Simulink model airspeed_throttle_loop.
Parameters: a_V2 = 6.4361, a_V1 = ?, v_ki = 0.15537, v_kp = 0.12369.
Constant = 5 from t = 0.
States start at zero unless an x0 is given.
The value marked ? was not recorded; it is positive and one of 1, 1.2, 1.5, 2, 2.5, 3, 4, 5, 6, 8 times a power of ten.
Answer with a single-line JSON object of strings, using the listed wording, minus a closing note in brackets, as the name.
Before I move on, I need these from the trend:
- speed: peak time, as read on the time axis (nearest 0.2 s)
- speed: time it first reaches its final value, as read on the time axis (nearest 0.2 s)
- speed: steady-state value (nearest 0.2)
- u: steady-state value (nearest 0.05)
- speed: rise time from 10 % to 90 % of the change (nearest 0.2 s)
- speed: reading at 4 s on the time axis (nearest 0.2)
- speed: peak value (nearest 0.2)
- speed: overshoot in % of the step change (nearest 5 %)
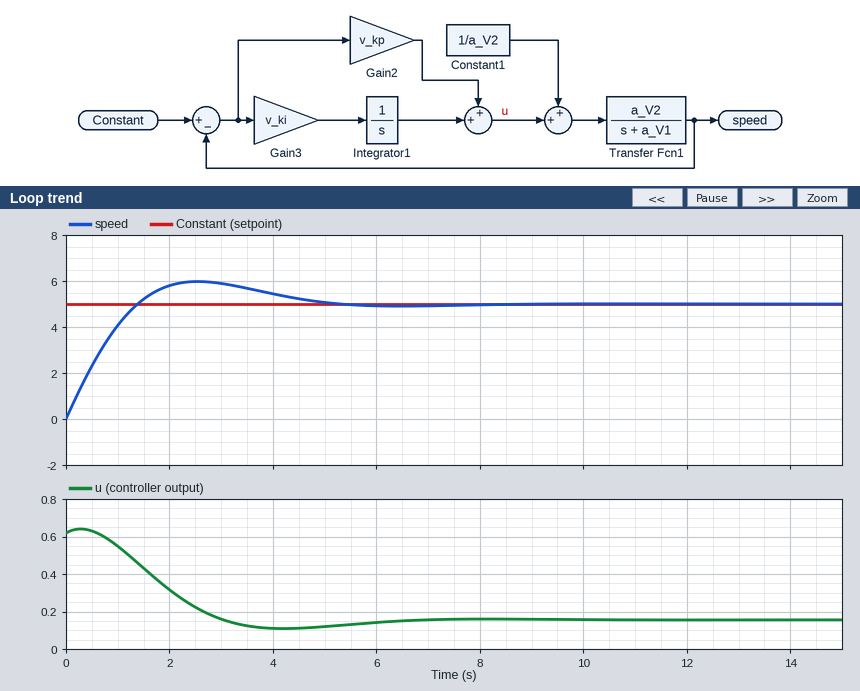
{"speed: peak time, as read on the time axis": "2.6 s", "speed: time it first reaches its final value, as read on the time axis": "1.4 s", "speed: steady-state value": "5.0", "u: steady-state value": "0.15", "speed: rise time from 10 % to 90 % of the change": "1.0 s", "speed: reading at 4 s on the time axis": "5.4", "speed: peak value": "6.0", "speed: overshoot in % of the step change": "20 %"}
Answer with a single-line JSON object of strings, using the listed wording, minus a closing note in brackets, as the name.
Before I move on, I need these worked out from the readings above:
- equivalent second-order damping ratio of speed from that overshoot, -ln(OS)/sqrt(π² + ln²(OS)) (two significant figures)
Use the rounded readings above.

{"equivalent second-order damping ratio of speed from that overshoot, -ln(OS)/sqrt(π² + ln²(OS))": "0.46"}
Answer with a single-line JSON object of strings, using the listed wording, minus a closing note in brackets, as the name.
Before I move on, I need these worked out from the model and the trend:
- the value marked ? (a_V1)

{"the value marked ?": "0.4"}
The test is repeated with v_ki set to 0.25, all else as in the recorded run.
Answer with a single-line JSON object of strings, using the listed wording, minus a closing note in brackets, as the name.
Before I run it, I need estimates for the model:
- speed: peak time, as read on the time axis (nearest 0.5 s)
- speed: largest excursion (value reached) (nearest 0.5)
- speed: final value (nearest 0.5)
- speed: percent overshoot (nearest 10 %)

{"speed: peak time, as read on the time axis": "2.0 s", "speed: largest excursion (value reached)": "6.5", "speed: final value": "5.0", "speed: percent overshoot": "30 %"}
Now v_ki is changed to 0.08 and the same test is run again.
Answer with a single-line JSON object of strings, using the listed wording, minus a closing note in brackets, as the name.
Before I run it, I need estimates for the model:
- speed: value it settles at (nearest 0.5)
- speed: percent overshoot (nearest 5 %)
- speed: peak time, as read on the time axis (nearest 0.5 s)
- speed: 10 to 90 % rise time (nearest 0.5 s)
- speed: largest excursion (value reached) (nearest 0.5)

{"speed: value it settles at": "5.0", "speed: percent overshoot": "10 %", "speed: peak time, as read on the time axis": "3.5 s", "speed: 10 to 90 % rise time": "1.5 s", "speed: largest excursion (value reached)": "5.5"}
